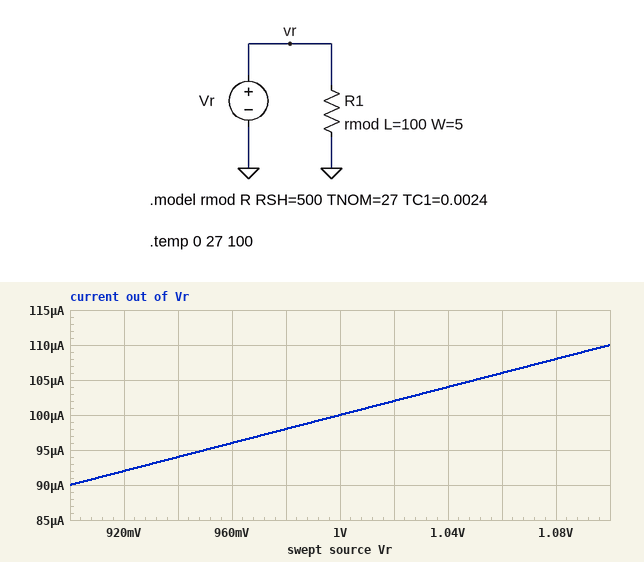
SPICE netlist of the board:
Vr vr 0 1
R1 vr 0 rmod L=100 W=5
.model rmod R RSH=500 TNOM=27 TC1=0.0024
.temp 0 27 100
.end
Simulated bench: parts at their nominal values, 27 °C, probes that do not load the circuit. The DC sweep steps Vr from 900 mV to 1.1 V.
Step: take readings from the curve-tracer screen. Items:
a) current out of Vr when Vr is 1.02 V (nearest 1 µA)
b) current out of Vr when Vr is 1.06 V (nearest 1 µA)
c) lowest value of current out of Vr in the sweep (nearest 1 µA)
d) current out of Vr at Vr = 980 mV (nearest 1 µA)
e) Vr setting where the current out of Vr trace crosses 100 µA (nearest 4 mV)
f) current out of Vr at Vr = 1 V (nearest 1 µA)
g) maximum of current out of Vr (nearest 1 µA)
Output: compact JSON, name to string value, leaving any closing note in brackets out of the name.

{"current out of Vr when Vr is 1.02 V": "102 µA", "current out of Vr when Vr is 1.06 V": "106 µA", "lowest value of current out of Vr in the sweep": "90 µA", "current out of Vr at Vr = 980 mV": "98 µA", "Vr setting where the current out of Vr trace crosses 100 µA": "1.000 V", "current out of Vr at Vr = 1 V": "100 µA", "maximum of current out of Vr": "110 µA"}
